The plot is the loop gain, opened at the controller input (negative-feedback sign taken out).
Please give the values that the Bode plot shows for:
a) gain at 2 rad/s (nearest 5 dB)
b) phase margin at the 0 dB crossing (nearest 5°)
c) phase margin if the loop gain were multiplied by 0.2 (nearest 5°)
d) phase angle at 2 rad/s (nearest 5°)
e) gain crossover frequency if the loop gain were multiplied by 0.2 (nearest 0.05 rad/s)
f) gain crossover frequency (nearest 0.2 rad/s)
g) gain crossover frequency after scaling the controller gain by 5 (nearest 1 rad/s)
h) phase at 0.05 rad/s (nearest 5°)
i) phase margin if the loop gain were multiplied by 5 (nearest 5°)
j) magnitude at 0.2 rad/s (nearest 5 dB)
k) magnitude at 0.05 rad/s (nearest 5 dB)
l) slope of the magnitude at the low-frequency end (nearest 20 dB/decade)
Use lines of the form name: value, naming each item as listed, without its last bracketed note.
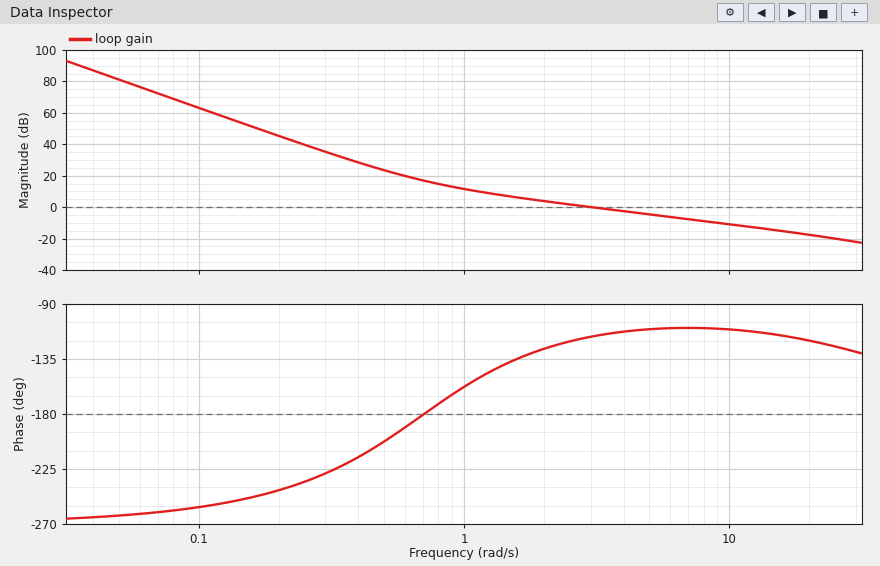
gain at 2 rad/s: 5 dB
phase margin at the 0 dB crossing: 65°
phase margin if the loop gain were multiplied by 0.2: 10°
phase angle at 2 rad/s: -125°
gain crossover frequency if the loop gain were multiplied by 0.2: 0.85 rad/s
gain crossover frequency: 3.0 rad/s
gain crossover frequency after scaling the controller gain by 5: 14 rad/s
phase at 0.05 rad/s: -265°
phase margin if the loop gain were multiplied by 5: 65°
magnitude at 0.2 rad/s: 45 dB
magnitude at 0.05 rad/s: 80 dB
slope of the magnitude at the low-frequency end: -60 dB/decade
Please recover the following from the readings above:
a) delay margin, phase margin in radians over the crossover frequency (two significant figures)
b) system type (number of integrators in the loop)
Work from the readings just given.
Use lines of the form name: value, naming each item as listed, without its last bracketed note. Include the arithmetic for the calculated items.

delay margin, phase margin in radians over the crossover frequency: 65 × π / 180 / 3 = 0.38 s
system type: 3
